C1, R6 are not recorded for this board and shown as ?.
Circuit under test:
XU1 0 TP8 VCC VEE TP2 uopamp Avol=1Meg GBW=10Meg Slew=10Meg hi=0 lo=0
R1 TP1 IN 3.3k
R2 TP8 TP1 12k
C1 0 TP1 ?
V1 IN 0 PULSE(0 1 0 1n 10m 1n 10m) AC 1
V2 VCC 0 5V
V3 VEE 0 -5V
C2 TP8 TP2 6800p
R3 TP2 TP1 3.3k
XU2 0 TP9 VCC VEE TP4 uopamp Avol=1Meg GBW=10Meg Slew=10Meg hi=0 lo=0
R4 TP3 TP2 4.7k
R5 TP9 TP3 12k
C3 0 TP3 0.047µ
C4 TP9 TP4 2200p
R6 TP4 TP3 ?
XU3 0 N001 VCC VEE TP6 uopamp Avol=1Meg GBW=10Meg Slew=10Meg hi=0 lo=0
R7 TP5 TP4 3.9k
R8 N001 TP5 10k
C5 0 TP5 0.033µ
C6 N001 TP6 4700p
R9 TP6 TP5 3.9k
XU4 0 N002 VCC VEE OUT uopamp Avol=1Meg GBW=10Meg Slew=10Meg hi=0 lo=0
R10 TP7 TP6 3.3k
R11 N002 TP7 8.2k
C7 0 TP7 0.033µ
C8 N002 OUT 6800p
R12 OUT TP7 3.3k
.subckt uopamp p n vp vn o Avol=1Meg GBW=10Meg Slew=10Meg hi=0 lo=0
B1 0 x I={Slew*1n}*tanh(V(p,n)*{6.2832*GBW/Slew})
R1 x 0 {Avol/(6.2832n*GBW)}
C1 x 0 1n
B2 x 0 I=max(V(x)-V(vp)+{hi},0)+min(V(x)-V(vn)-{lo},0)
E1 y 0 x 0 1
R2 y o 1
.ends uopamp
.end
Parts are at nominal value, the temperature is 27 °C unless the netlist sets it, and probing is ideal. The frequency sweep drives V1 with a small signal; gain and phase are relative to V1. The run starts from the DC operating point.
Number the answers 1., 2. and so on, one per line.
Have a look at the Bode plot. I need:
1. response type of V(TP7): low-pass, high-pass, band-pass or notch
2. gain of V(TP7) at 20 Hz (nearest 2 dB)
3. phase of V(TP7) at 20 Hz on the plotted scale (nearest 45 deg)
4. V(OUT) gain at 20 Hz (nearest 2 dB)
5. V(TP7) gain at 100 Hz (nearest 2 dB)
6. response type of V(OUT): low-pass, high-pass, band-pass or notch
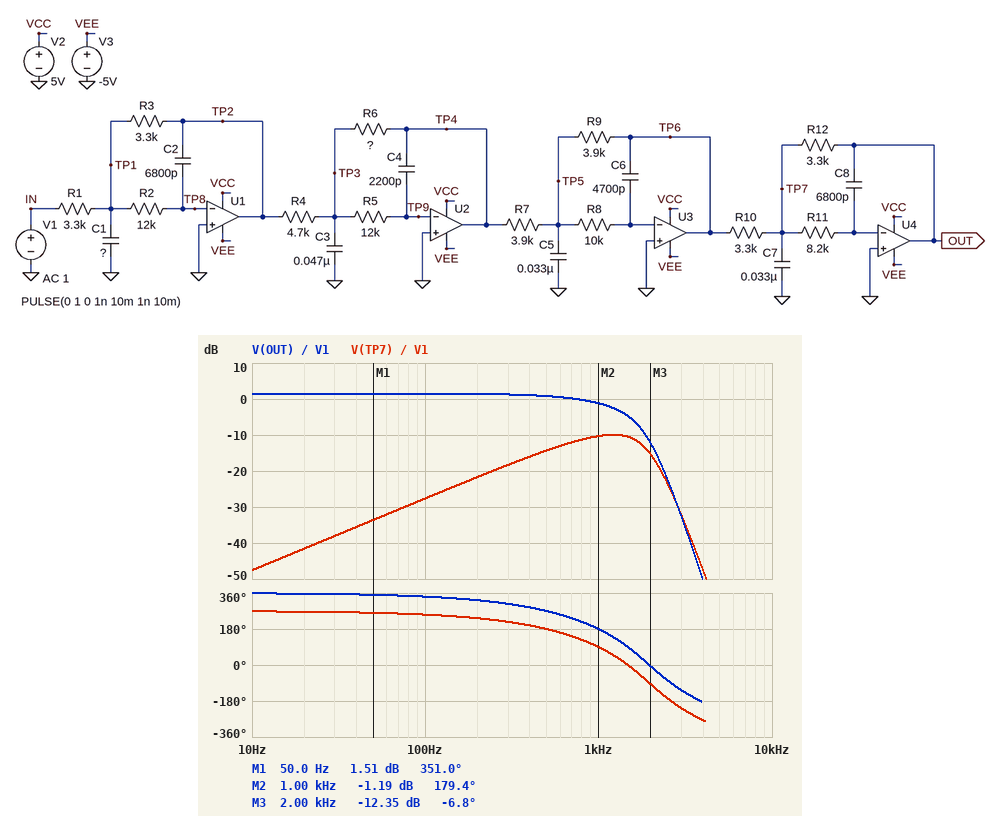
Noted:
1. band-pass
2. -42 dB
3. 270 deg
4. 2 dB
5. -28 dB
6. low-pass
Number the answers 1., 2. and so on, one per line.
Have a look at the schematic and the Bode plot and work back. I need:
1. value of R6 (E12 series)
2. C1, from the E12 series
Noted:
1. 5.6 kΩ
2. 27 nF
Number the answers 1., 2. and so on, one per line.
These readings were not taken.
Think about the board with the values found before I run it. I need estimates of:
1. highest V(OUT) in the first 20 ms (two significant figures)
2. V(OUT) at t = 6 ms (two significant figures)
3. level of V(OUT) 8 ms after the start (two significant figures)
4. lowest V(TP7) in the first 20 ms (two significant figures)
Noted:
1. 1.2 V
2. 540 mV
3. 300 mV
4. -190 mV
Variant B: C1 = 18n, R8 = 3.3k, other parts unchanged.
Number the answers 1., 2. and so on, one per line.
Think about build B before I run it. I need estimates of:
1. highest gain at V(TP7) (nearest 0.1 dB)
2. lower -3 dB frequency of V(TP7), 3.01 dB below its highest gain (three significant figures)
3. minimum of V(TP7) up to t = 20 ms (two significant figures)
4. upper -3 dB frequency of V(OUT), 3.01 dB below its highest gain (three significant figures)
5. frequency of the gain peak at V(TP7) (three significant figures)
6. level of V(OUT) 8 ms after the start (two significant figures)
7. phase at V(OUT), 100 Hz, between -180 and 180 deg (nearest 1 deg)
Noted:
1. -9.0 dB
2. 701 Hz
3. -210 mV
4. 1.13 kHz
5. 1.41 kHz
6. 290 mV
7. -16 deg
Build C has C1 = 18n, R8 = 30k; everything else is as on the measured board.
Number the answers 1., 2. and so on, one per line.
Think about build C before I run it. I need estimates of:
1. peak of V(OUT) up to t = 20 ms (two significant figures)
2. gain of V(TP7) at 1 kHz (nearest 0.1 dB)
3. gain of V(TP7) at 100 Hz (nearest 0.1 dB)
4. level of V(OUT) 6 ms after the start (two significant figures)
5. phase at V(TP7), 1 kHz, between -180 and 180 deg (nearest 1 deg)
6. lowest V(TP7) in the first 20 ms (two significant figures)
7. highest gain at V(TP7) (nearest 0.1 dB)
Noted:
1. 1.1 V
2. -15.9 dB
3. -27.7 dB
4. 560 mV
5. 54 deg
6. -120 mV
7. -15.5 dB
